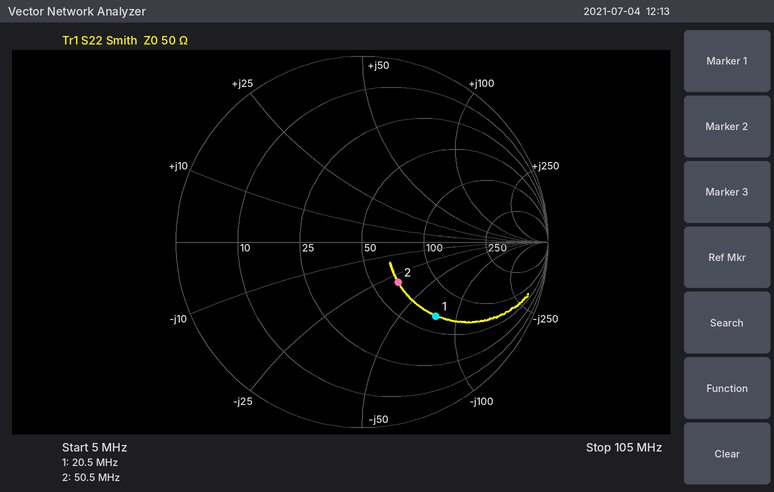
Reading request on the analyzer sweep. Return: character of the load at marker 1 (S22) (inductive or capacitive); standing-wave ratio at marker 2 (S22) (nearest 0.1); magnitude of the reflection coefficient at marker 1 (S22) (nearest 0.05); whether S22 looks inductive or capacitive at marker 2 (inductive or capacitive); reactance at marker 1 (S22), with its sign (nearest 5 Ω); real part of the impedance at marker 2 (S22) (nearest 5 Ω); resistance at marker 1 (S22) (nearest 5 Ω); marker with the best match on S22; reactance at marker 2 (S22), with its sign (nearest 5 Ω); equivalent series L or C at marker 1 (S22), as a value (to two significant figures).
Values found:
capacitive
1.8
0.55
capacitive
-75 Ω
65 Ω
65 Ω
marker 2
-30 Ω
100 pF
